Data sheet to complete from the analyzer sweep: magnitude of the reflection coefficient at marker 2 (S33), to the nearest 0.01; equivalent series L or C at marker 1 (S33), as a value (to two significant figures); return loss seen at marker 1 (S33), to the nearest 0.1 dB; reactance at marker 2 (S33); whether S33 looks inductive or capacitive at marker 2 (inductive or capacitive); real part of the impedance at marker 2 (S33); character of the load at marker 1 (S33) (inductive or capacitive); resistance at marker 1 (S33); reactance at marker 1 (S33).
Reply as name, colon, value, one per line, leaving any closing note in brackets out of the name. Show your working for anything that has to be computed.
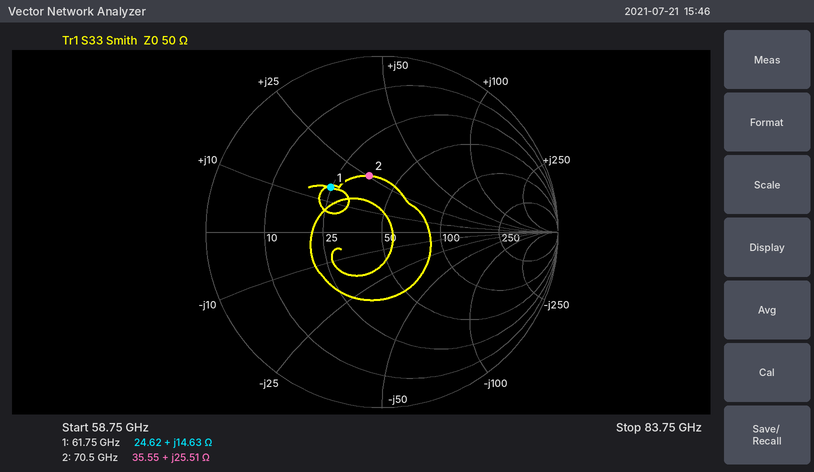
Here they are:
magnitude of the reflection coefficient at marker 2 (S33), to the nearest 0.01: 0.33
equivalent series L or C at marker 1 (S33), as a value: L = 14.63 Ω/(2π × 61.75 GHz) ≈ 38 pH
return loss seen at marker 1 (S33), to the nearest 0.1 dB: 8.3 dB
reactance at marker 2: +25.51 Ω
whether S33 looks inductive or capacitive at marker 2: inductive
real part of the impedance at marker 2: 35.55 Ω
character of the load at marker 1 (S33): inductive
resistance at marker 1: 24.62 Ω
reactance at marker 1: +14.63 Ω
